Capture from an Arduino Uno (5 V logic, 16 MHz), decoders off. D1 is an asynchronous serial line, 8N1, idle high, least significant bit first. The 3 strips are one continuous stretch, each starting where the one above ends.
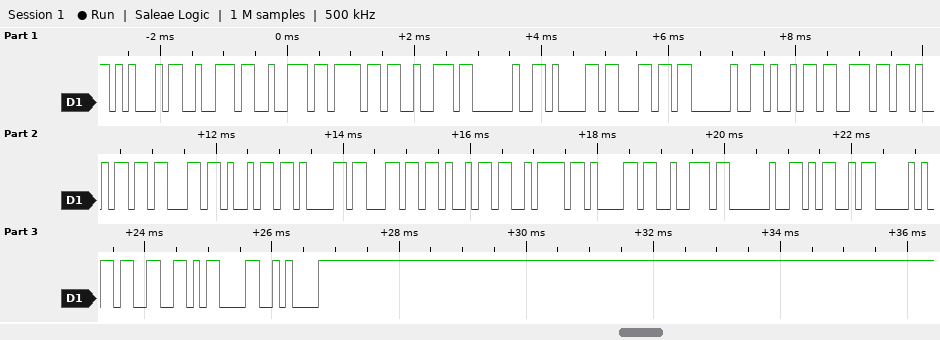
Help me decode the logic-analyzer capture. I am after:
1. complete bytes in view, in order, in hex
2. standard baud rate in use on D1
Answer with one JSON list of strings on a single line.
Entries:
["0x45 0x72 0x72 0x6F 0x72 0x20 0x61 0x6C 0x20 0x69 0x6E 0x69 0x63 0x69 0x61 0x6C 0x69 0x7A 0x61 0x72 0x20 0x4D 0x50 0x33 0x0D 0x0A", "9600 baud"]
